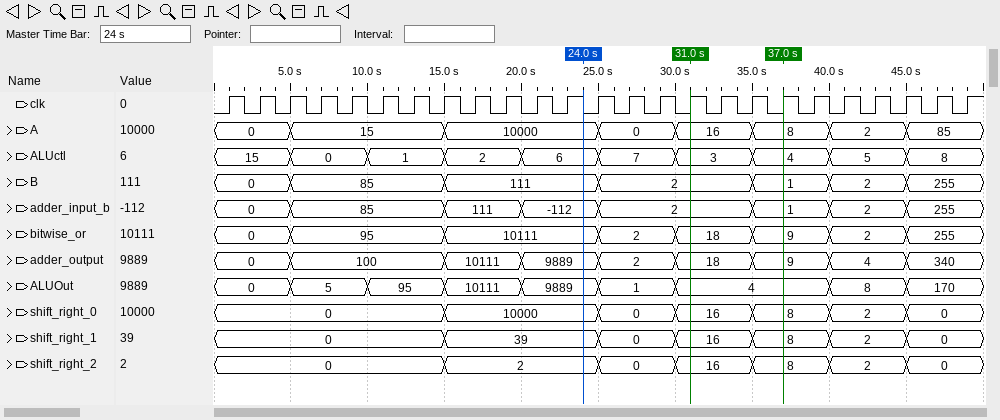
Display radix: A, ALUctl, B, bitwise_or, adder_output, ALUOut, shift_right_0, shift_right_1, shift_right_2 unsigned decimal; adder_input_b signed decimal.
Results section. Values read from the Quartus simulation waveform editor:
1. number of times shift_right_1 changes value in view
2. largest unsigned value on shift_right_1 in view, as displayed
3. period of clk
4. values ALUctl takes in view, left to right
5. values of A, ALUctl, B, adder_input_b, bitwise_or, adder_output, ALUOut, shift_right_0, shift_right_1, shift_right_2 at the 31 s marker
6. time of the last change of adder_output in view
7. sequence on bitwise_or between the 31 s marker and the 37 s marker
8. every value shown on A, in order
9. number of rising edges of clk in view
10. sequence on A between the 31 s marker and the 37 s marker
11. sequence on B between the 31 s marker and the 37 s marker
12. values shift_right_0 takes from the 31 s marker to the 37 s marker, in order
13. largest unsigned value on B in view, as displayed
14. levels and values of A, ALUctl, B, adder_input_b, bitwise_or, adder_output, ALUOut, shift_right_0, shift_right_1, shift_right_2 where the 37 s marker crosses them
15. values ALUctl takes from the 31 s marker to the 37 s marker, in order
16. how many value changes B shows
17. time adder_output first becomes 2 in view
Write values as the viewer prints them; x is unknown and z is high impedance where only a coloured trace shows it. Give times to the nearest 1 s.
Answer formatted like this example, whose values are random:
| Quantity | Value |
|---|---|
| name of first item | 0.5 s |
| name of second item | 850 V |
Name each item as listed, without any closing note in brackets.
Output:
| Quantity | Value |
|---|---|
| number of times shift_right_1 changes value in view | 6 |
| largest unsigned value on shift_right_1 in view, as displayed | 39 |
| period of clk | 2 s |
| values ALUctl takes in view, left to right | 15, 0, 1, 2, 6, 7, 3, 4, 5, 8 |
| values of A, ALUctl, B, adder_input_b, bitwise_or, adder_output, ALUOut, shift_right_0, shift_right_1, shift_right_2 at the 31 s marker | A=16, ALUctl=3, B=2, adder_input_b=2, bitwise_or=18, adder_output=18, ALUOut=4, shift_right_0=16, shift_right_1=16, shift_right_2=16 |
| time of the last change of adder_output in view | 45 s |
| sequence on bitwise_or between the 31 s marker and the 37 s marker | 18, 9 |
| every value shown on A, in order | 0, 15, 10000, 0, 16, 8, 2, 85 |
| number of rising edges of clk in view | 25 |
| sequence on A between the 31 s marker and the 37 s marker | 16, 8 |
| sequence on B between the 31 s marker and the 37 s marker | 2, 1 |
| values shift_right_0 takes from the 31 s marker to the 37 s marker, in order | 16, 8 |
| largest unsigned value on B in view, as displayed | 255 |
| levels and values of A, ALUctl, B, adder_input_b, bitwise_or, adder_output, ALUOut, shift_right_0, shift_right_1, shift_right_2 where the 37 s marker crosses them | A=8, ALUctl=4, B=1, adder_input_b=1, bitwise_or=9, adder_output=9, ALUOut=4, shift_right_0=8, shift_right_1=8, shift_right_2=8 |
| values ALUctl takes from the 31 s marker to the 37 s marker, in order | 3, 4 |
| how many value changes B shows | 6 |
| time adder_output first becomes 2 in view | 25 s |
